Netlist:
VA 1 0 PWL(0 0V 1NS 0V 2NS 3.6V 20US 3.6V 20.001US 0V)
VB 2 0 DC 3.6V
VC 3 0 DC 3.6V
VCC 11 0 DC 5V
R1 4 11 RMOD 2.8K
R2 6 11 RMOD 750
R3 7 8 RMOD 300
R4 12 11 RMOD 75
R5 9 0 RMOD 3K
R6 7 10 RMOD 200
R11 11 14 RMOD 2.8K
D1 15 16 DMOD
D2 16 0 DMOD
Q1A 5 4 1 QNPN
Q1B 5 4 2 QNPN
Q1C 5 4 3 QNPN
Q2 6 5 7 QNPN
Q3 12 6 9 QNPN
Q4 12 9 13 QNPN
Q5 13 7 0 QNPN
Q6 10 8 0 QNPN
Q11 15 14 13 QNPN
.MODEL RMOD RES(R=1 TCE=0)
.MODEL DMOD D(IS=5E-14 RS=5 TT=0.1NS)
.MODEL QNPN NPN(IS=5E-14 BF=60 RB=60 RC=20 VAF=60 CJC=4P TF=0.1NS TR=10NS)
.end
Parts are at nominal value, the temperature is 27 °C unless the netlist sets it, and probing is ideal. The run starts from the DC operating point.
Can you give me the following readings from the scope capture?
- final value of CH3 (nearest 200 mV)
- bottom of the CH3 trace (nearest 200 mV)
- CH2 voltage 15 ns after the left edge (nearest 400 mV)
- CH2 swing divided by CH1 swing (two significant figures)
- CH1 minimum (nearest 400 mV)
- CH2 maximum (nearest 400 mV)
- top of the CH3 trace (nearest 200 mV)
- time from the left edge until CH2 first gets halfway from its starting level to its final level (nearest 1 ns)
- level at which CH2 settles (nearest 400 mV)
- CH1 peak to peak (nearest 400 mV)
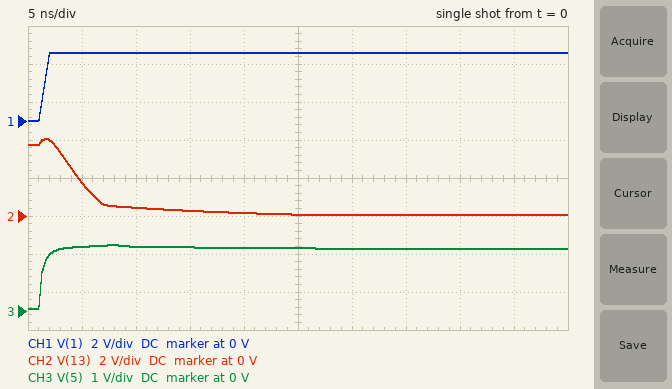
1.6 V
0 V
400 mV
1.1
0 V
4.0 V
1.8 V
5 ns
0 V
3.6 V
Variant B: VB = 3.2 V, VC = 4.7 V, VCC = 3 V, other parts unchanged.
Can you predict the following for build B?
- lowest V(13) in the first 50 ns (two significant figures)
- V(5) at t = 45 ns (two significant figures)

45 mV
1.4 V
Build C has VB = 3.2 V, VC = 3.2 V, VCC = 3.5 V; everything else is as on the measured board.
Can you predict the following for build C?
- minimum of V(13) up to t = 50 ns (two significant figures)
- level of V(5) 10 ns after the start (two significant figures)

46 mV
1.5 V
